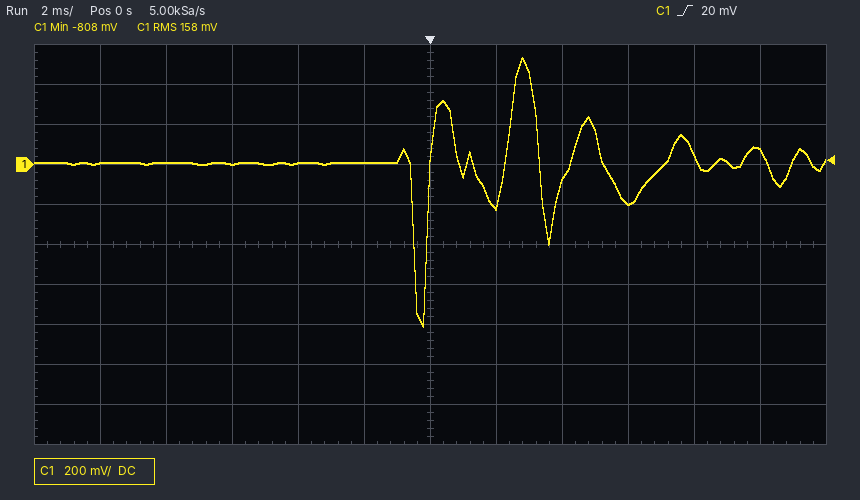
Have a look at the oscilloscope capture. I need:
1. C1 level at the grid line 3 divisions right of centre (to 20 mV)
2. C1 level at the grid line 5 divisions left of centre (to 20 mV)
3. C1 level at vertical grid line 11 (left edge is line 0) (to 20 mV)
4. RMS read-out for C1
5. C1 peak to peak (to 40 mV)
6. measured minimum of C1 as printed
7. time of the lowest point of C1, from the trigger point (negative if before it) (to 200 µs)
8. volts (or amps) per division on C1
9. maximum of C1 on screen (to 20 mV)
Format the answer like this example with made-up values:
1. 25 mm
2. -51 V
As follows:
1. -200 mV
2. 0 mV
3. 60 mV
4. 158 mV
5. 1.36 V
6. -808 mV
7. -200 µs
8. 200 mV
9. 540 mV
